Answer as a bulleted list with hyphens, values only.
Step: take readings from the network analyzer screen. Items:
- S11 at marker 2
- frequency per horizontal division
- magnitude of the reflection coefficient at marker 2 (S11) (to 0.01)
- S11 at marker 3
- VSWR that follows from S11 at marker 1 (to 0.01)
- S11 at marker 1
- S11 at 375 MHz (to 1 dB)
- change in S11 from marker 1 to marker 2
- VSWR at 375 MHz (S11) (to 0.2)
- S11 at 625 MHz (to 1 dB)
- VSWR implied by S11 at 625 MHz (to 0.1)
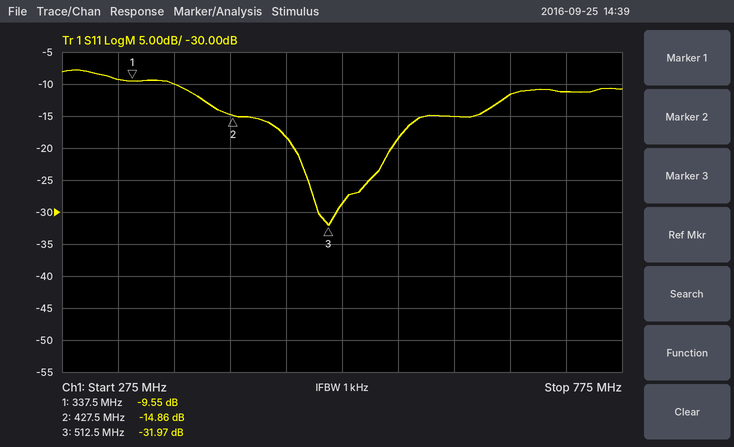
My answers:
- -14.86 dB
- 50 MHz
- 0.18
- -31.97 dB
- 2.00
- -9.55 dB
- -10 dB
- -5.31 dB
- 2.0
- -15 dB
- 1.4
